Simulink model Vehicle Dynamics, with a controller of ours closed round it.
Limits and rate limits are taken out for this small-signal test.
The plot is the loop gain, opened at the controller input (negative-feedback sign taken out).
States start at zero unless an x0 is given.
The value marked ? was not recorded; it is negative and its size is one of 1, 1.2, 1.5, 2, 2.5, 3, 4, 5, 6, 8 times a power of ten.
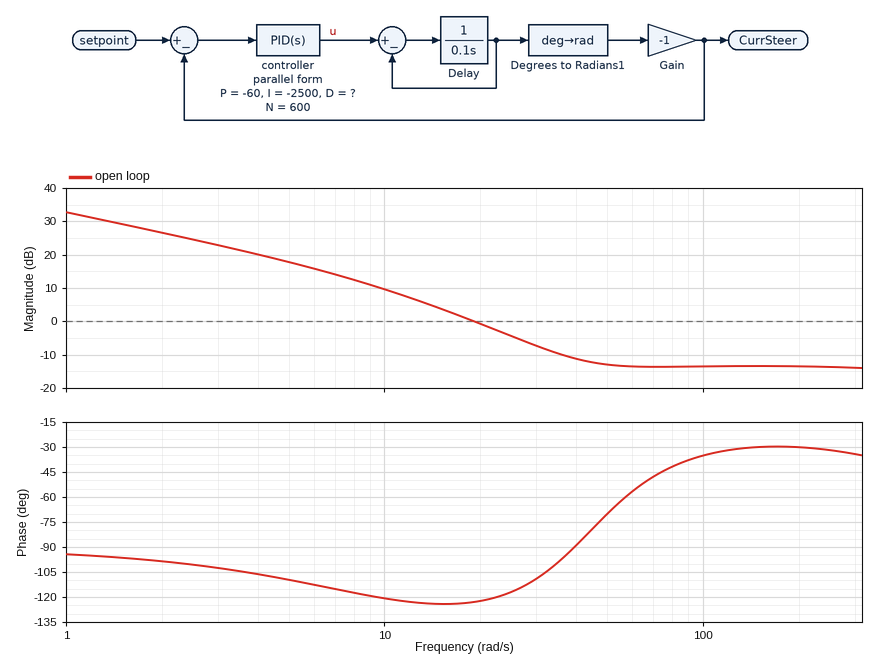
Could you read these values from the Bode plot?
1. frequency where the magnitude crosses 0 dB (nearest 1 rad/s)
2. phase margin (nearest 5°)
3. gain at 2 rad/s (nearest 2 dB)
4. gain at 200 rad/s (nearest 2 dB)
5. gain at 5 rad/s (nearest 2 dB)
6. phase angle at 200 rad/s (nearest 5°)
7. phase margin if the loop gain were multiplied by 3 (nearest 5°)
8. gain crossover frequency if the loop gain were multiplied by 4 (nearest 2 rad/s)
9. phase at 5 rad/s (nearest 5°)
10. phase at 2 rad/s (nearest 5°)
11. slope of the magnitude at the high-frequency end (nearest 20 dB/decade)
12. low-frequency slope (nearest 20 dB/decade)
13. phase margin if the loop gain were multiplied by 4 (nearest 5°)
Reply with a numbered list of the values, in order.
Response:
1. 19 rad/s
2. 55°
3. 26 dB
4. -14 dB
5. 18 dB
6. -30°
7. 80°
8. 44 rad/s
9. -110°
10. -100°
11. 0 dB/decade
12. -20 dB/decade
13. 100°
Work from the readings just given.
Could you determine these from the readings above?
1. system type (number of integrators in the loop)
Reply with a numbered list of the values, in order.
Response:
1. 1
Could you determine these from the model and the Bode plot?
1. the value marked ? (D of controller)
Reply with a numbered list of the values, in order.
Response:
1. -1.2
